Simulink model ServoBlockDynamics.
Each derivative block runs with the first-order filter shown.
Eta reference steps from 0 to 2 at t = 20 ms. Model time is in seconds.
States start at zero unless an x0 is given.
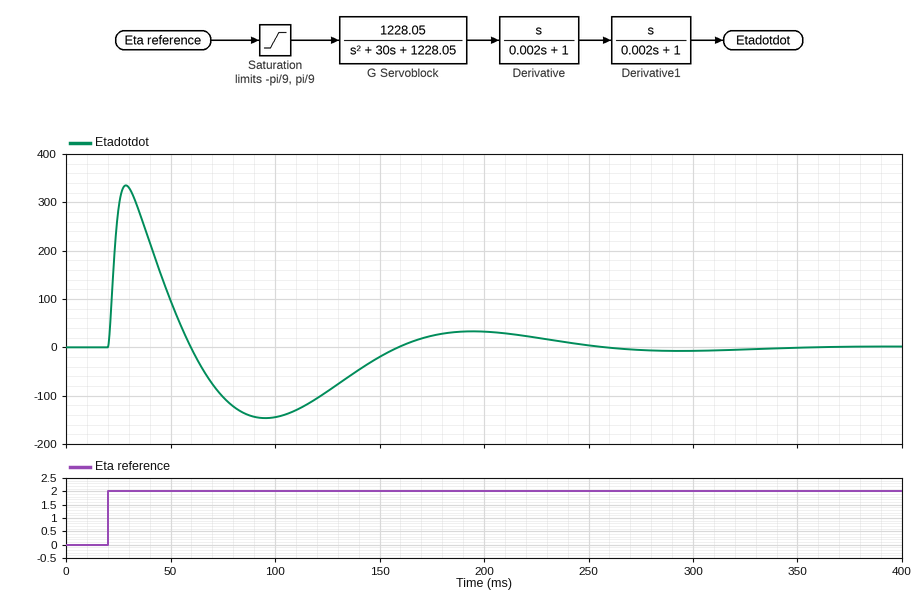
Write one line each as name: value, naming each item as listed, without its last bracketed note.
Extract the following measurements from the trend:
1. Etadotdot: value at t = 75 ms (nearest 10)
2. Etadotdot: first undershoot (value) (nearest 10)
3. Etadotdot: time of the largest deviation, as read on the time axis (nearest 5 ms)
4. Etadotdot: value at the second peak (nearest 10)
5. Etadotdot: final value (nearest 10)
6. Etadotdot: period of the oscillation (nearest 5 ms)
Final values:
Etadotdot: value at t = 75 ms: -100
Etadotdot: first undershoot (value): -150
Etadotdot: time of the largest deviation, as read on the time axis: 30 ms
Etadotdot: value at the second peak: 30
Etadotdot: final value: 0
Etadotdot: period of the oscillation: 165 ms
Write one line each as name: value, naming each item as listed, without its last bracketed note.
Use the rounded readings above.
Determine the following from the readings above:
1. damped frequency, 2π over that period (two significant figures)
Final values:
damped frequency, 2π over that period: 0.038 rad/ms
